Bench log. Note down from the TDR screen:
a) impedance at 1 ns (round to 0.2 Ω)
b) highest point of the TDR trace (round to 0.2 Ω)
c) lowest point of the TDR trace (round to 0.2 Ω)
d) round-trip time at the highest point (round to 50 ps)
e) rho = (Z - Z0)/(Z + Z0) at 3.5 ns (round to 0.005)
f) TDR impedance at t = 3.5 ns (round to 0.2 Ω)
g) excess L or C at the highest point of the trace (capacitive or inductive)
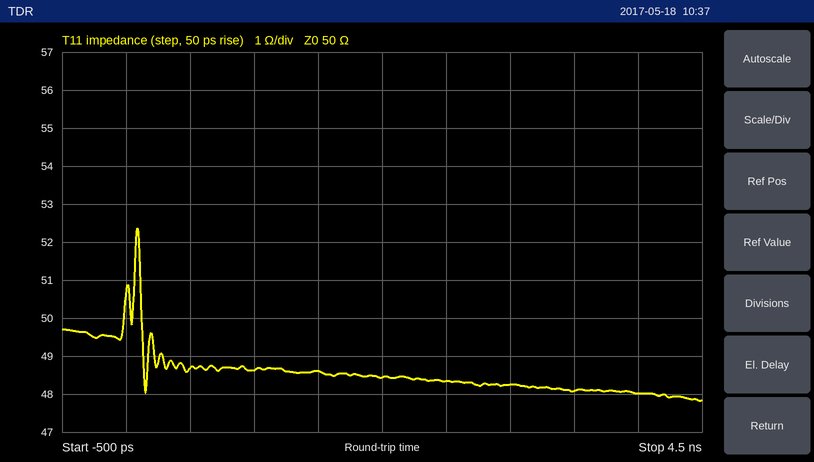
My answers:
48.6 Ω
52.4 Ω
47.8 Ω
100 ps
-0.020
48.0 Ω
inductive
